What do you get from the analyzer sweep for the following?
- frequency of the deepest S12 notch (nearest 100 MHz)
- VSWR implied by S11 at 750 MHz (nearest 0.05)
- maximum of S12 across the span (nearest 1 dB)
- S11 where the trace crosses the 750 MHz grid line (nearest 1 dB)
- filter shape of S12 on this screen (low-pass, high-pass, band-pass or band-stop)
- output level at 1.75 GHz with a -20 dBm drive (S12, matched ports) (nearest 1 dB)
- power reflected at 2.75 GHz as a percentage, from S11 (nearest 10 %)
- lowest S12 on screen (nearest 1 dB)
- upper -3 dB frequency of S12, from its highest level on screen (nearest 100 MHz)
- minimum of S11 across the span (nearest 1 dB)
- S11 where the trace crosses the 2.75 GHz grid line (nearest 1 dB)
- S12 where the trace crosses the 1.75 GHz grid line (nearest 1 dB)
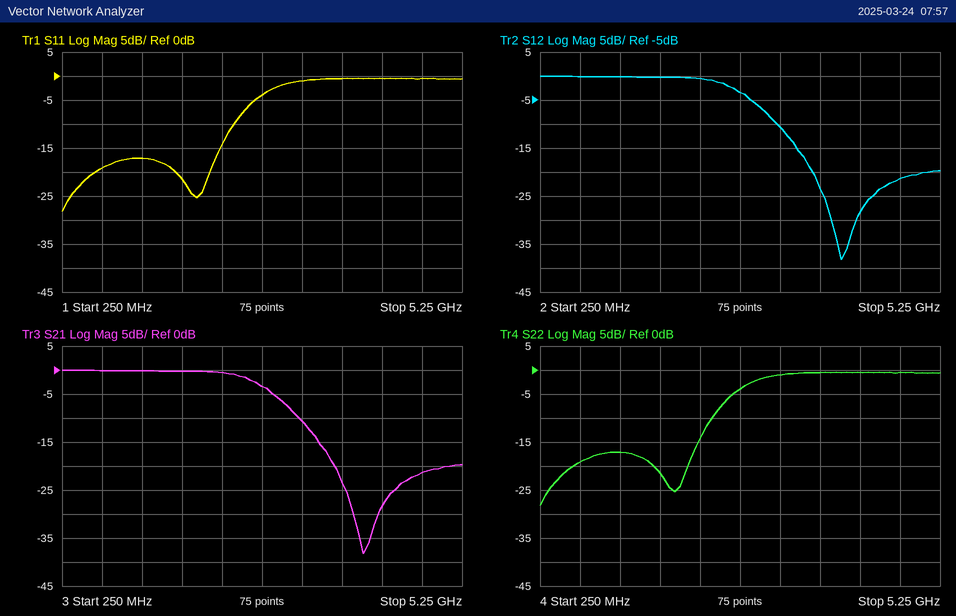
4.0 GHz
1.25
0 dB
-19 dB
low-pass
-20 dBm
40 %
-38 dB
2.7 GHz
-28 dB
-4 dB
0 dB
